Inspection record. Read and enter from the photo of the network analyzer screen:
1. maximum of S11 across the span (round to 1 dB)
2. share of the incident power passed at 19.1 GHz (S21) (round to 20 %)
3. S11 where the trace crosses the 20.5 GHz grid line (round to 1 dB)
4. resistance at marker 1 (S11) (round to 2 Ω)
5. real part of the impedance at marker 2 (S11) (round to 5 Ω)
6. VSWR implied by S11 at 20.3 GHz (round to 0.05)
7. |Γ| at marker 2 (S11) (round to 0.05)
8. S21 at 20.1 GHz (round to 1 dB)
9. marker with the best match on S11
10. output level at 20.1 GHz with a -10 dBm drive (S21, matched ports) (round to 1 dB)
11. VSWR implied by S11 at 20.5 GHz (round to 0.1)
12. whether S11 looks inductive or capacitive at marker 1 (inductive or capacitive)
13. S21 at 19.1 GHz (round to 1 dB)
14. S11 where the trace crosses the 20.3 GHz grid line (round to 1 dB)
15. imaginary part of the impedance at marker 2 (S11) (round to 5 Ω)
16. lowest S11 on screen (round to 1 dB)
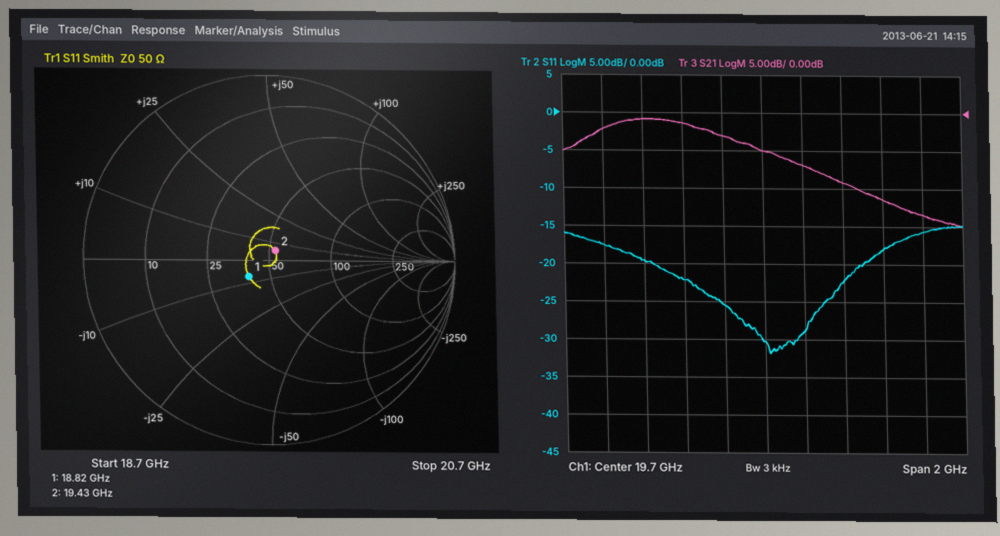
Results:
-15 dB
80 %
-16 dB
40 Ω
55 Ω
1.30
0.05
-9 dB
marker 2
-19 dBm
1.4
capacitive
-1 dB
-18 dB
+5 Ω
-32 dB
